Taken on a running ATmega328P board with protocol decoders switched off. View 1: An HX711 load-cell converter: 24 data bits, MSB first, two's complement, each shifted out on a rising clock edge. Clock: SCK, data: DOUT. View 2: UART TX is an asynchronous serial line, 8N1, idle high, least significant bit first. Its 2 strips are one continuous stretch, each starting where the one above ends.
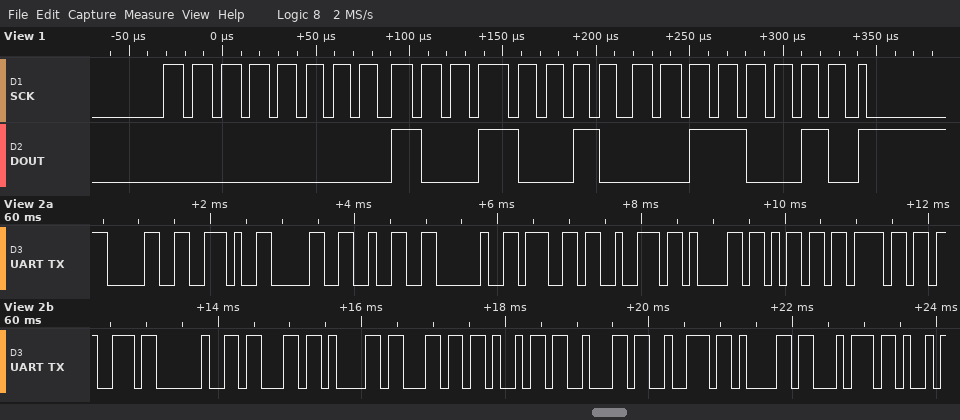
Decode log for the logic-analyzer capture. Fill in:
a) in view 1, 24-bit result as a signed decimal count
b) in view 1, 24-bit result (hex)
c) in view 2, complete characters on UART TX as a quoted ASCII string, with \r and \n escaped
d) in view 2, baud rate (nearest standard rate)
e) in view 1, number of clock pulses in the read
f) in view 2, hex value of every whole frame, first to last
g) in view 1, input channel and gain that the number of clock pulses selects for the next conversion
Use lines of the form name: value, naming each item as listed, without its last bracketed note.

in view 1, 24-bit result as a signed decimal count: 37426
in view 1, 24-bit result: 0x009232
in view 2, complete characters on UART TX as a quoted ASCII string, with \r and \n escaped: "0.02 gramos calibrat"
in view 2, baud rate: 9600 baud
in view 1, number of clock pulses in the read: 25
in view 2, hex value of every whole frame, first to last: 30 2E 30 32 20 67 72 61 6D 6F 73 20 63 61 6C 69 62 72 61 74
in view 1, input channel and gain that the number of clock pulses selects for the next conversion: channel A, gain 128
